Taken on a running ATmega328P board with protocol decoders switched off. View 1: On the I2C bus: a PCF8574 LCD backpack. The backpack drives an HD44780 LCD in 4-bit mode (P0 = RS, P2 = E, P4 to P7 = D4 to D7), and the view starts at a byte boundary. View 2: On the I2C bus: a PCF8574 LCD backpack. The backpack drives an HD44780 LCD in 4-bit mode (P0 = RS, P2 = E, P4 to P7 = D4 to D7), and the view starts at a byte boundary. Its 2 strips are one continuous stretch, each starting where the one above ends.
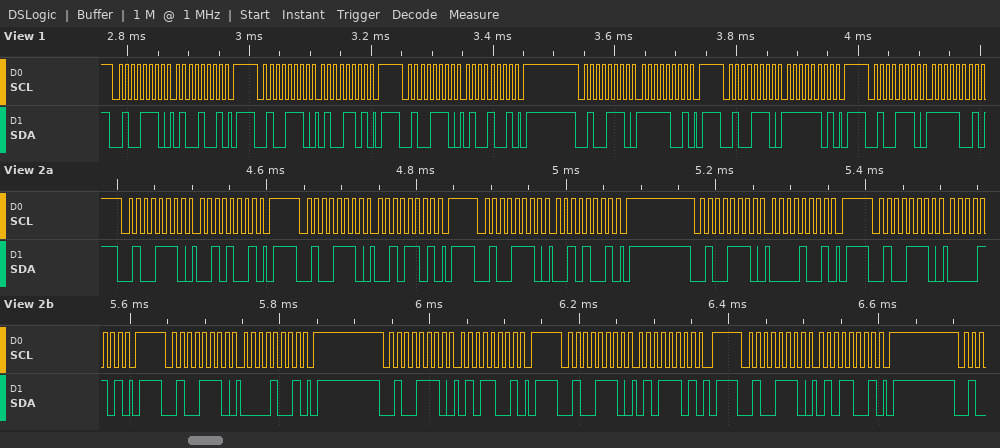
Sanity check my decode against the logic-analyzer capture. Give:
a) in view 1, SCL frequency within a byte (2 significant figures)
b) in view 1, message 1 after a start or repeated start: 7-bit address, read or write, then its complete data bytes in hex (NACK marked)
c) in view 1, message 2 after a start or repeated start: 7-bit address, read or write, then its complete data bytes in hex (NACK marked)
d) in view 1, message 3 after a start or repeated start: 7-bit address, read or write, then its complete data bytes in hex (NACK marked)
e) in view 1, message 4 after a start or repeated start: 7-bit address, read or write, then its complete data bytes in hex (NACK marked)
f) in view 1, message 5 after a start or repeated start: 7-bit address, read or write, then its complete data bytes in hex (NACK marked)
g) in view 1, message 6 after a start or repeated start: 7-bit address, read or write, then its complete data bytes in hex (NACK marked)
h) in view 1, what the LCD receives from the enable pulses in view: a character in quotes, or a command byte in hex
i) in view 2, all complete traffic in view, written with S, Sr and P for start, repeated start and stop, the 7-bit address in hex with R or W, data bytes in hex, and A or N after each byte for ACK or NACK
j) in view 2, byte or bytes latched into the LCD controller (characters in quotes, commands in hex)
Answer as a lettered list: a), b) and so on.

a) 100 kHz
b) 0x27 write: 49
c) 0x27 write: 4D
d) 0x27 write: 49
e) 0x27 write: F9
f) 0x27 write: FD
g) 0x27 write: F9
h) 'O'
i) S 27W A 29 A P S 27W A 2D A P S 27W A 29 A P S 27W A 09 A P S 27W A 0D A P S 27W A 09 A P S 27W A 59 A P S 27W A 5D A P S 27W A 59 A P
j) ' '
